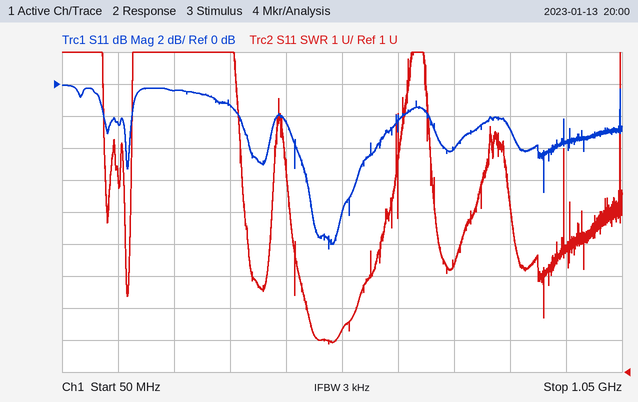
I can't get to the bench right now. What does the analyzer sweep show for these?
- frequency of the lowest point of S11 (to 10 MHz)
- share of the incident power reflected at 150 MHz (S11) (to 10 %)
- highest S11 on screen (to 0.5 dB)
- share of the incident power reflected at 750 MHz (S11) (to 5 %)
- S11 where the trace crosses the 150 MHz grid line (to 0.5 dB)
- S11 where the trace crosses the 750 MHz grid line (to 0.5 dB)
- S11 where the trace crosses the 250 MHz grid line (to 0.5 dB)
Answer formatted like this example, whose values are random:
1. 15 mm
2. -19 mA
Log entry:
1. 530 MHz
2. 60 %
3. 0.0 dB
4. 40 %
5. -2.5 dB
6. -4.0 dB
7. -0.5 dB
